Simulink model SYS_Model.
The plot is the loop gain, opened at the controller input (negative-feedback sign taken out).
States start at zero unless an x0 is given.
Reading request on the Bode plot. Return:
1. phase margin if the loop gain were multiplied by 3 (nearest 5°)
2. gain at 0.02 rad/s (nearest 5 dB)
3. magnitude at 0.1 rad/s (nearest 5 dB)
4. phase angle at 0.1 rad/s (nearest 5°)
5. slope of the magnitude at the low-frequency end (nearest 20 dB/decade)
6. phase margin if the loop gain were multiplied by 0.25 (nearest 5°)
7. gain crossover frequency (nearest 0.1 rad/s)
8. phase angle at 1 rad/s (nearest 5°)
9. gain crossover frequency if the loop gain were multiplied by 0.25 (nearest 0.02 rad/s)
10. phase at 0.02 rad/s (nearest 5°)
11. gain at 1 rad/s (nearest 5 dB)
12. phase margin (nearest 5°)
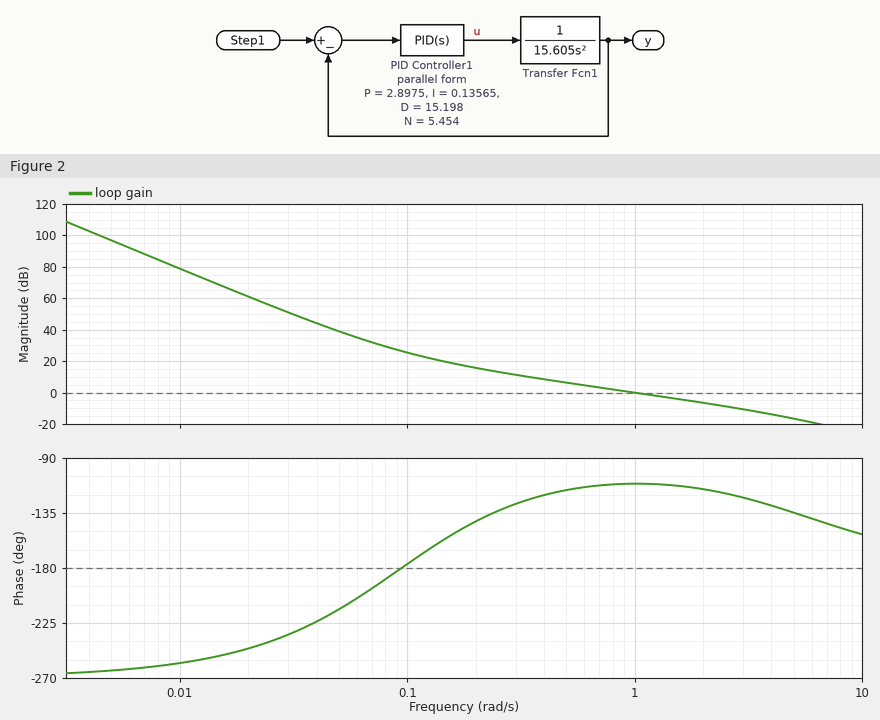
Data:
60°
60 dB
25 dB
-175°
-60 dB/decade
50°
1.0 rad/s
-110°
0.28 rad/s
-245°
0 dB
70°
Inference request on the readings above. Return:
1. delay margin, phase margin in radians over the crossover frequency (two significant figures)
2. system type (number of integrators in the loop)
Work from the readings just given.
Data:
1.2 s
3
